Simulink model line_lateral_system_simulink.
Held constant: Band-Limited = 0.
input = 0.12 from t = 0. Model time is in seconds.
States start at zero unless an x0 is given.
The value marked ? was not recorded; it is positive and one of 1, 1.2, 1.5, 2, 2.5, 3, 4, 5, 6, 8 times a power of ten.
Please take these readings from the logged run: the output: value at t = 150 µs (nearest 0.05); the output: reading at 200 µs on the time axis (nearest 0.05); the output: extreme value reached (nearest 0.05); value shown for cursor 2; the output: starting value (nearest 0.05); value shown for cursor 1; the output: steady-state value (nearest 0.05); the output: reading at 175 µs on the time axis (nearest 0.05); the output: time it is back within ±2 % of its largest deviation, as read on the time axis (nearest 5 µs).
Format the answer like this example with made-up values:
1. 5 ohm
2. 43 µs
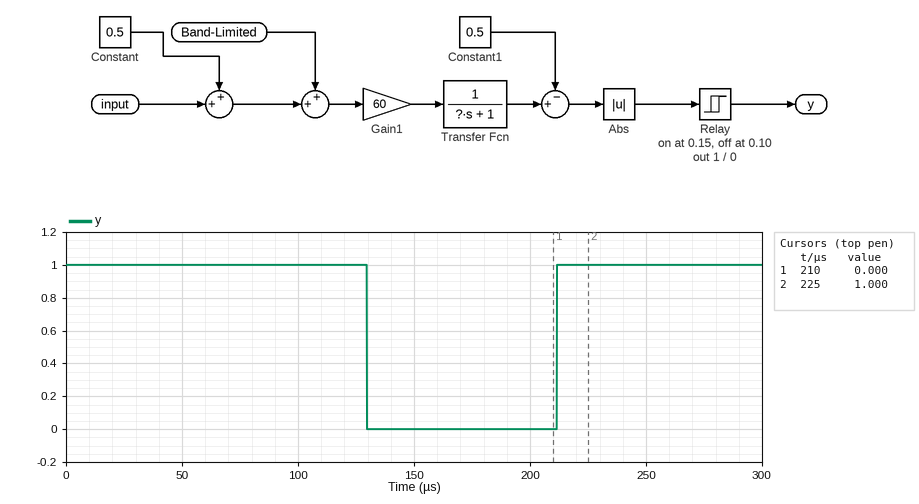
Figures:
1. 0.00
2. 0.00
3. 0.00
4. 1.000
5. 1.00
6. 0.000
7. 1.00
8. 0.00
9. 210 µs
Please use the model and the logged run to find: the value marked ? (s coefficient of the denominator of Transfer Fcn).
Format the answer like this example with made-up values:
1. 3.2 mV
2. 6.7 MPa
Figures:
1. 0.012
